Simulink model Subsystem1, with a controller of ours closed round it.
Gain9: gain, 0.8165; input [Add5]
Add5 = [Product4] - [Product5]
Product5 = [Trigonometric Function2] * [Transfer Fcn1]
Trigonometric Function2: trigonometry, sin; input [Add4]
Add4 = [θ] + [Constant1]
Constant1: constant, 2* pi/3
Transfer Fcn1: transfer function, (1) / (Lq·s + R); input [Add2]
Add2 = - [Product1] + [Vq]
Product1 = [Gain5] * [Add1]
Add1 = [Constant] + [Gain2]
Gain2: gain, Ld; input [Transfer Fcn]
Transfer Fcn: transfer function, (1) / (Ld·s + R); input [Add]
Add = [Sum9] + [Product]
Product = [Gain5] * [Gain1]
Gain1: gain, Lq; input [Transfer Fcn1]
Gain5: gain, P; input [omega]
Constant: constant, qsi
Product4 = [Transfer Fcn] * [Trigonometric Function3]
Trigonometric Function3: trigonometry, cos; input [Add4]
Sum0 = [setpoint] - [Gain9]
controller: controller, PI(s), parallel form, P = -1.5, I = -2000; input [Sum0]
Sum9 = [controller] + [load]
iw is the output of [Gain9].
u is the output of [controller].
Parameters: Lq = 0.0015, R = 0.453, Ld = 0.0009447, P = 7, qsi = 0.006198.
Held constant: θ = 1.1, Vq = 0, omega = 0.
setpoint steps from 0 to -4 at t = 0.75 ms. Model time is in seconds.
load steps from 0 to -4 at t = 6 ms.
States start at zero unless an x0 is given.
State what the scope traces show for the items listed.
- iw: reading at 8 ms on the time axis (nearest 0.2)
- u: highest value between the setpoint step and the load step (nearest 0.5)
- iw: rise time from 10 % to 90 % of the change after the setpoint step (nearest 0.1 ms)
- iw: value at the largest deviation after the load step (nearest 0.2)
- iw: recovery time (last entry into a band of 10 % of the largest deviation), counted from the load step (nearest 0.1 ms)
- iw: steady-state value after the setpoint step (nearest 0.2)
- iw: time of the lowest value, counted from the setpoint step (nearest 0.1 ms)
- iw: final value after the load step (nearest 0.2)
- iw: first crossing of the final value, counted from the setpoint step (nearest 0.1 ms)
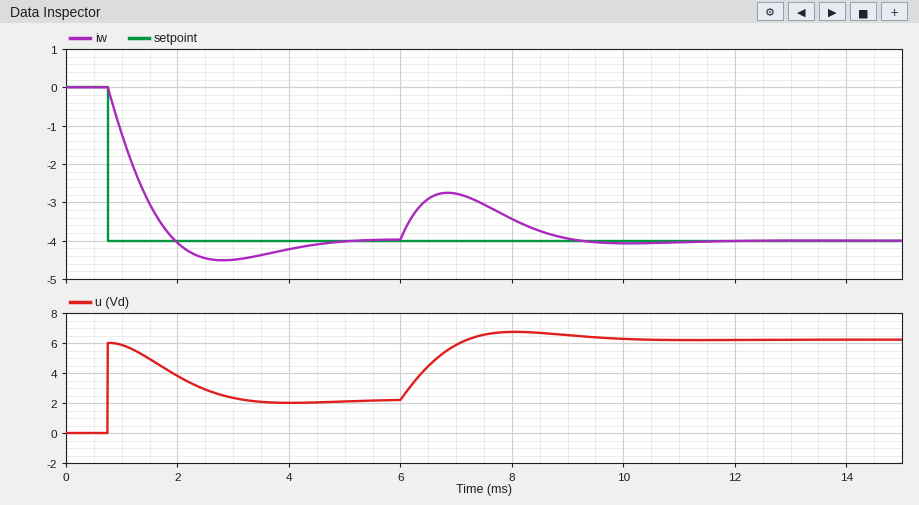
-3.4
6.0
0.9 ms
-2.8
2.8 ms
-4.0
2.1 ms
-4.0
1.2 ms
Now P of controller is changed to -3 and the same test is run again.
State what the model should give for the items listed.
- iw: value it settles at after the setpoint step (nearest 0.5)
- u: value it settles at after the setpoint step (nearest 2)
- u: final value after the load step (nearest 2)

-4.0
2
6
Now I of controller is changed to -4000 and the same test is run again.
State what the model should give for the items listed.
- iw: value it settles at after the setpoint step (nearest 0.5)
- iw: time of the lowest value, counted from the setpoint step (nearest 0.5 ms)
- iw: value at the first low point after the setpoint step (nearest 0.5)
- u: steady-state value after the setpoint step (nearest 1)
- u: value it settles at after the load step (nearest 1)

-4.0
1.5 ms
-5.0
2
6
